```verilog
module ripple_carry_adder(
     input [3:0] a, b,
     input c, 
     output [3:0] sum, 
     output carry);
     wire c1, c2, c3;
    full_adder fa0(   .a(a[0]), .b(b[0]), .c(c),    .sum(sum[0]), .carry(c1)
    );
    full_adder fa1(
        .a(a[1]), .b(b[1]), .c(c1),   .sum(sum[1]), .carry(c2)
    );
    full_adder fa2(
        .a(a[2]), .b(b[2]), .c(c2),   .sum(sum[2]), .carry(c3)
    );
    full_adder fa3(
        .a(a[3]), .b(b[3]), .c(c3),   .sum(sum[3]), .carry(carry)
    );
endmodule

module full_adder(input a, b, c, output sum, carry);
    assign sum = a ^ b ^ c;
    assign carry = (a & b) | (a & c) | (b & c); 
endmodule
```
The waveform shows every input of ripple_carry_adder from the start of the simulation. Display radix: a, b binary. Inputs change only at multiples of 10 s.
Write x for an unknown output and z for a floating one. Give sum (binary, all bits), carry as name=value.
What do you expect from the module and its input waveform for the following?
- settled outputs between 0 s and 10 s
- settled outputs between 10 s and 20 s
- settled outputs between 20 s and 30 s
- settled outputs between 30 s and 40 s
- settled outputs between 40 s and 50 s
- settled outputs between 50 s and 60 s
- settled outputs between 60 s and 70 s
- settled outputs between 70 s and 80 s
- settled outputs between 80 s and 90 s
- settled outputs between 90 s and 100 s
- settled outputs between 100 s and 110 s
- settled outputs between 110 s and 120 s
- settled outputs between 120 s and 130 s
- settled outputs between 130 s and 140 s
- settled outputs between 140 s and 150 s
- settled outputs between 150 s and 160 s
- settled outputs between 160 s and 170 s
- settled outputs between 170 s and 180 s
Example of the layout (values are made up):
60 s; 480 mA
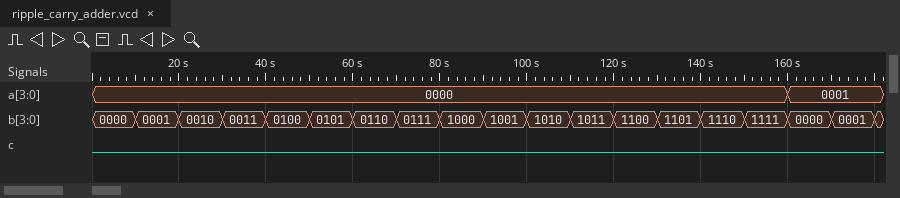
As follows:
sum=0000, carry=0; sum=0001, carry=0; sum=0010, carry=0; sum=0011, carry=0; sum=0100, carry=0; sum=0101, carry=0; sum=0110, carry=0; sum=0111, carry=0; sum=1000, carry=0; sum=1001, carry=0; sum=1010, carry=0; sum=1011, carry=0; sum=1100, carry=0; sum=1101, carry=0; sum=1110, carry=0; sum=1111, carry=0; sum=0001, carry=0; sum=0010, carry=0
